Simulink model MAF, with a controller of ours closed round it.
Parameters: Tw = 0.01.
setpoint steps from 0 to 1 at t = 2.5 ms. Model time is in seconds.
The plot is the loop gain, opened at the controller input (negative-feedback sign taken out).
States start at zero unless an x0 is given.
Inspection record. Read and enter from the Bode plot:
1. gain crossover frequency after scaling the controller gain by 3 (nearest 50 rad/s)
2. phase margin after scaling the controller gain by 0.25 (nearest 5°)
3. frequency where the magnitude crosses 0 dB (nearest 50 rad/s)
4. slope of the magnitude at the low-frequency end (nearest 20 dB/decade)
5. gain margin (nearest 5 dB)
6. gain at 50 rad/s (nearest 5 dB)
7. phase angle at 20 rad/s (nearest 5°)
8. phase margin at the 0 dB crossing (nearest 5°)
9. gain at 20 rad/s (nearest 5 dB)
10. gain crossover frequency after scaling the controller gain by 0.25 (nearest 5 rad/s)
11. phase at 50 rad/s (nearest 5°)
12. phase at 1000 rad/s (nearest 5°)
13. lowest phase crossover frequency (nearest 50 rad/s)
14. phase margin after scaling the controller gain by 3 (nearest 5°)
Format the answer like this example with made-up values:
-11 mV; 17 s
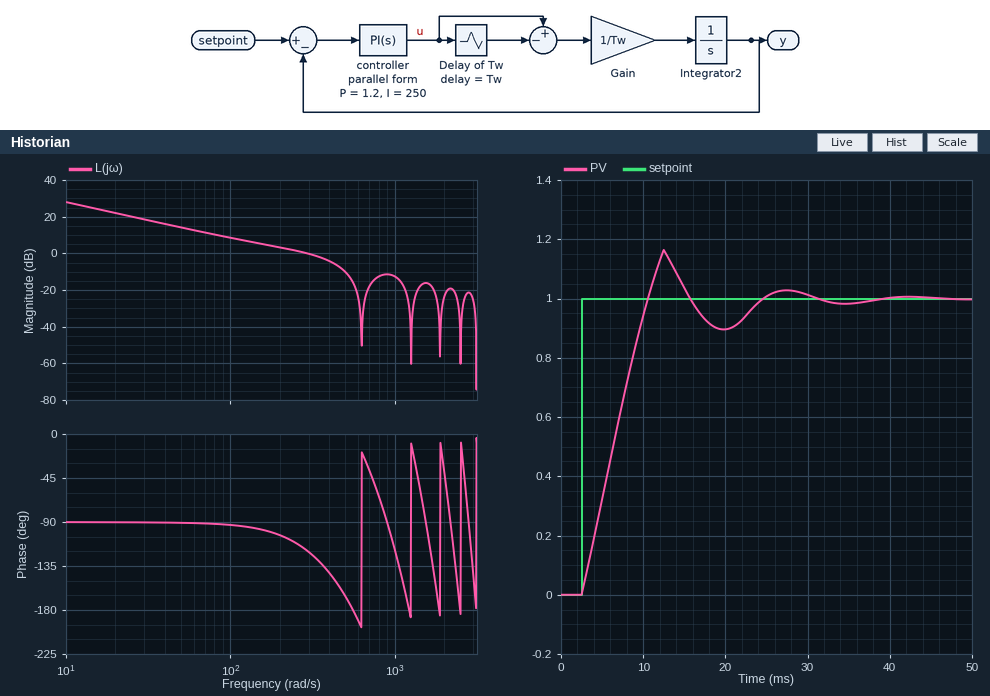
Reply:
500 rad/s; 90°; 300 rad/s; -20 dB/decade; 15 dB; 15 dB; -90°; 60°; 20 dB; 65 rad/s; -90°; -120°; 550 rad/s; 15°
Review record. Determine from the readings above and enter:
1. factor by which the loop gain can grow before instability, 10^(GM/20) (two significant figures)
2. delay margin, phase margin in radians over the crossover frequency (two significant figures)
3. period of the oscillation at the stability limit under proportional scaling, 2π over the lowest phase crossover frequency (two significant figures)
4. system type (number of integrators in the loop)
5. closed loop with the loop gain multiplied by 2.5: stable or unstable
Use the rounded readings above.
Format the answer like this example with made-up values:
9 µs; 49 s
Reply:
5.6; 0.0035 s; 0.011 s; 1; stable
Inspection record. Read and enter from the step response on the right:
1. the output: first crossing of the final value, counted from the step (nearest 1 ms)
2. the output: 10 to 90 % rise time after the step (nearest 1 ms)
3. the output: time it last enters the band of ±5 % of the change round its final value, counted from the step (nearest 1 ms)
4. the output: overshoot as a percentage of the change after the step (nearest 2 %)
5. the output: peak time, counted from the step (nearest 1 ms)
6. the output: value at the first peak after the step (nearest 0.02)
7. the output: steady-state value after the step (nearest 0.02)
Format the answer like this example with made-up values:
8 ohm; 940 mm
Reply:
8 ms; 6 ms; 20 ms; 16 %; 10 ms; 1.16; 1.00
